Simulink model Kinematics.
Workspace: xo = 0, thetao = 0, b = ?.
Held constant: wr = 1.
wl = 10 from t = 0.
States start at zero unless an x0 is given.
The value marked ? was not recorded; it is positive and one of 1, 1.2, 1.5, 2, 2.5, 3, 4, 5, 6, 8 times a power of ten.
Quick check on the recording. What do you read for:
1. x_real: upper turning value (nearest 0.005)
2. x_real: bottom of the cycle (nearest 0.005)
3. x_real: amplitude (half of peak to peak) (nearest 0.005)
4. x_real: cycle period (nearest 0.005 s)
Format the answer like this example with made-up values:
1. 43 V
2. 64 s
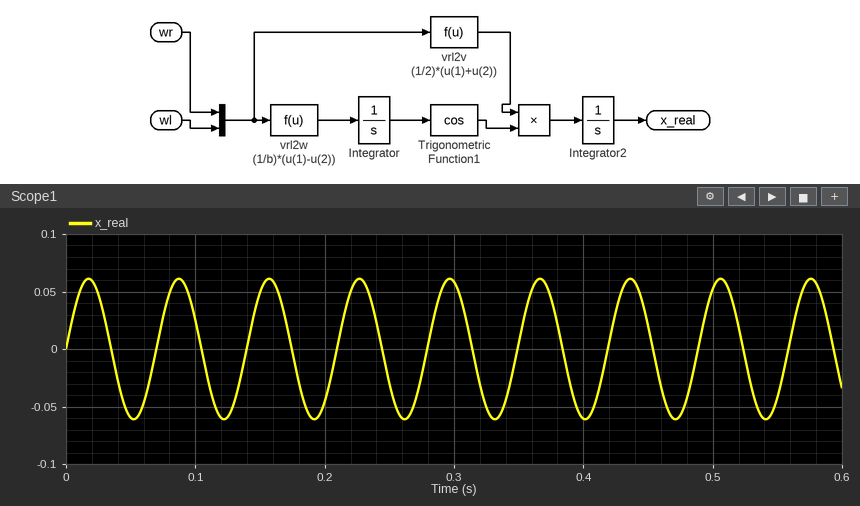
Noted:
1. 0.060
2. -0.060
3. 0.060
4. 0.070 s
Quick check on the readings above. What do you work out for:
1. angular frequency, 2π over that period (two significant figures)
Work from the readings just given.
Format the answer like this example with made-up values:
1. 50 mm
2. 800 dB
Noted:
1. 90 rad/s
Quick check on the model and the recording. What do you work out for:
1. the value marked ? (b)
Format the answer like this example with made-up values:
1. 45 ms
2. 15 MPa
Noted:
1. 0.1
